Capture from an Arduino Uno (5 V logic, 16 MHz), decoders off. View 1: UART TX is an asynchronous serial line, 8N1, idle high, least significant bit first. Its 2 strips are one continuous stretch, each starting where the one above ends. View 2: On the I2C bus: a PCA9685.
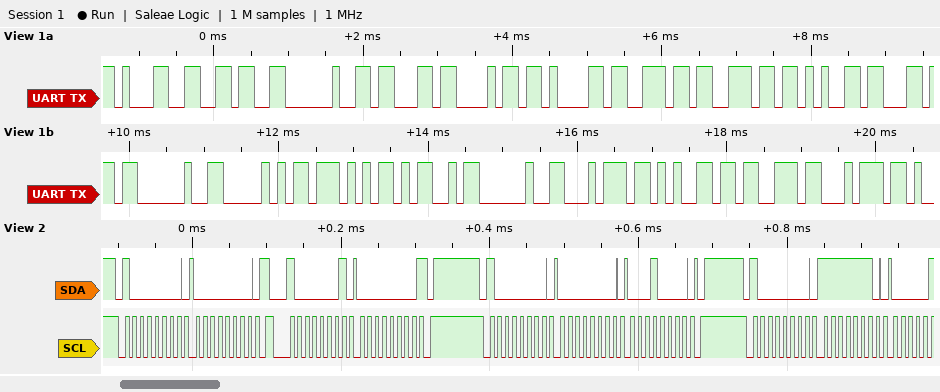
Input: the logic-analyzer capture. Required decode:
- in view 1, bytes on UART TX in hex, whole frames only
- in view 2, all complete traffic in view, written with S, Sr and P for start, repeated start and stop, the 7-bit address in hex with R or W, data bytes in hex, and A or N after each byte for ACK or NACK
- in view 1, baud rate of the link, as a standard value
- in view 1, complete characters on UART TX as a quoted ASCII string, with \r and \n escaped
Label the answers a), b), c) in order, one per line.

a) 0x31 0x36 0x20 0x63 0x68 0x61 0x6E 0x6E 0x65 0x6C 0x20 0x50 0x57 0x4D 0x20 0x74 0x65 0x73 0x74
b) S 40W A 00 A Sr 40R A 00 N P S 40W A 00 A 10 A P S 40W A FE A
c) 9600 baud
d) "16 channel PWM test"
